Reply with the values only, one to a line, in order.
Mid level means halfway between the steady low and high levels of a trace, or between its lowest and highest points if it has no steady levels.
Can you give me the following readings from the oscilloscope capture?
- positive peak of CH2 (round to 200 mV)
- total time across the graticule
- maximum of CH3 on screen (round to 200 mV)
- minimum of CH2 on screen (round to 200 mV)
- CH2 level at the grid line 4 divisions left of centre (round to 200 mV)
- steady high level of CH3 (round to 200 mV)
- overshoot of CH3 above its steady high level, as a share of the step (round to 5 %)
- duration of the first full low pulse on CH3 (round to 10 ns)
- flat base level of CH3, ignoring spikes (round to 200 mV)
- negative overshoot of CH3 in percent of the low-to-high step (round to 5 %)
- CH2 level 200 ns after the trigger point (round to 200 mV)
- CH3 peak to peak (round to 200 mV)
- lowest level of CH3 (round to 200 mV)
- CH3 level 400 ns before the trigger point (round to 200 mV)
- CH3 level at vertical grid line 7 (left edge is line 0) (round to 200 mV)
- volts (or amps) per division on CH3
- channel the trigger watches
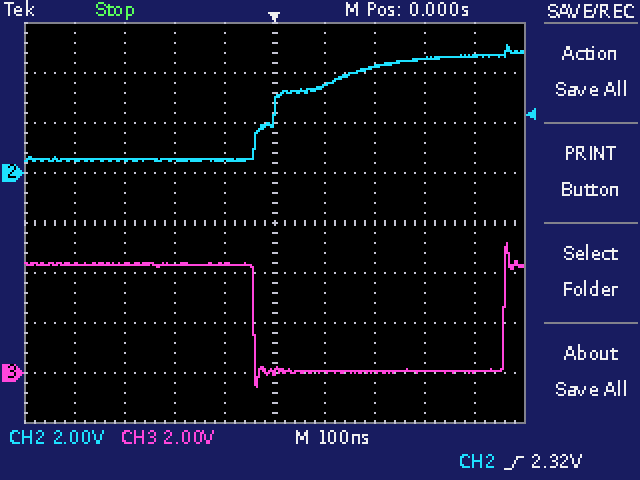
5.2 V
1 µs
5.2 V
400 mV
600 mV
4.4 V
20 %
500 ns
0.0 V
15 %
4.2 V
5.8 V
-600 mV
4.4 V
0.0 V
2 V
CH2
